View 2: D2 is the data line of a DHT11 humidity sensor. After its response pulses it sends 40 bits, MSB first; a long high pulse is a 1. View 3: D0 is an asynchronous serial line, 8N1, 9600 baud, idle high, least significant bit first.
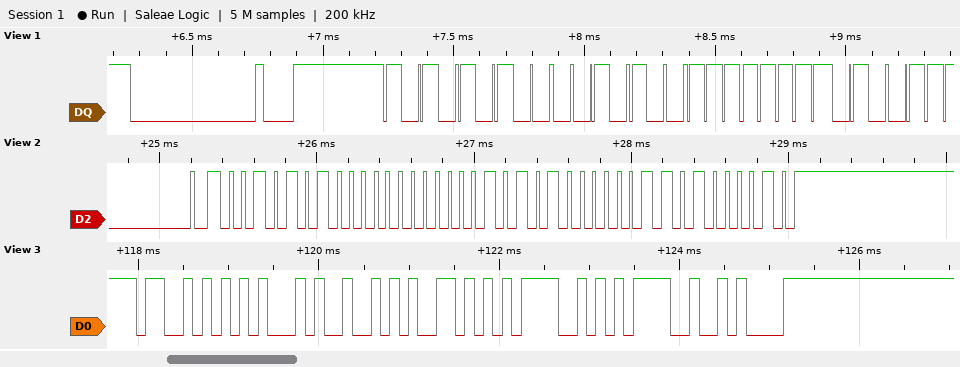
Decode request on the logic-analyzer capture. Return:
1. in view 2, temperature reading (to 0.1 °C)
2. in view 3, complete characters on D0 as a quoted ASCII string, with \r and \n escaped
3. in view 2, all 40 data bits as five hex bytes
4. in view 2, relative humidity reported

21.3 °C
"SERVO=\n"
2A 00 15 03 42
42 %
